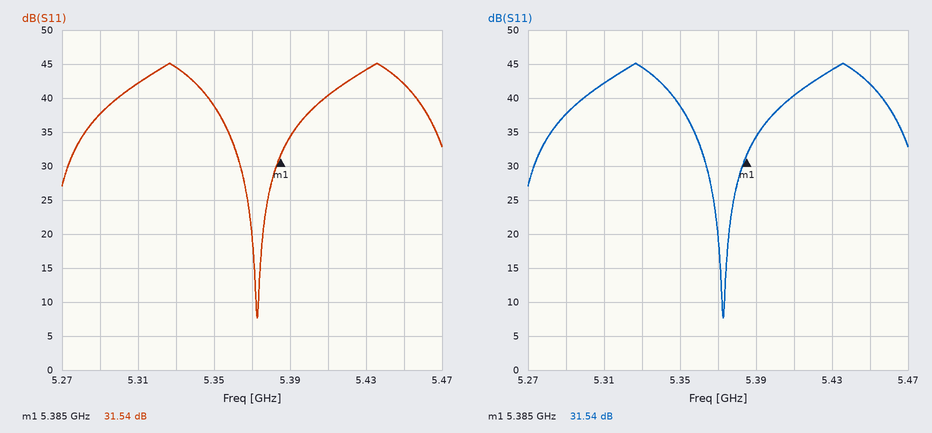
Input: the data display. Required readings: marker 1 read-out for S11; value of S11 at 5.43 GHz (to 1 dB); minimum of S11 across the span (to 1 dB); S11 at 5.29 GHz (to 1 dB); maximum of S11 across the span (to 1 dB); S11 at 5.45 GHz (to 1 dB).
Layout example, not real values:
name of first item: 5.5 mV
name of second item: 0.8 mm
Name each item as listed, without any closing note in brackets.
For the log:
marker 1 read-out for S11: 31.54 dB
value of S11 at 5.43 GHz: 44 dB
minimum of S11 across the span: 8 dB
S11 at 5.29 GHz: 38 dB
maximum of S11 across the span: 45 dB
S11 at 5.45 GHz: 42 dB
